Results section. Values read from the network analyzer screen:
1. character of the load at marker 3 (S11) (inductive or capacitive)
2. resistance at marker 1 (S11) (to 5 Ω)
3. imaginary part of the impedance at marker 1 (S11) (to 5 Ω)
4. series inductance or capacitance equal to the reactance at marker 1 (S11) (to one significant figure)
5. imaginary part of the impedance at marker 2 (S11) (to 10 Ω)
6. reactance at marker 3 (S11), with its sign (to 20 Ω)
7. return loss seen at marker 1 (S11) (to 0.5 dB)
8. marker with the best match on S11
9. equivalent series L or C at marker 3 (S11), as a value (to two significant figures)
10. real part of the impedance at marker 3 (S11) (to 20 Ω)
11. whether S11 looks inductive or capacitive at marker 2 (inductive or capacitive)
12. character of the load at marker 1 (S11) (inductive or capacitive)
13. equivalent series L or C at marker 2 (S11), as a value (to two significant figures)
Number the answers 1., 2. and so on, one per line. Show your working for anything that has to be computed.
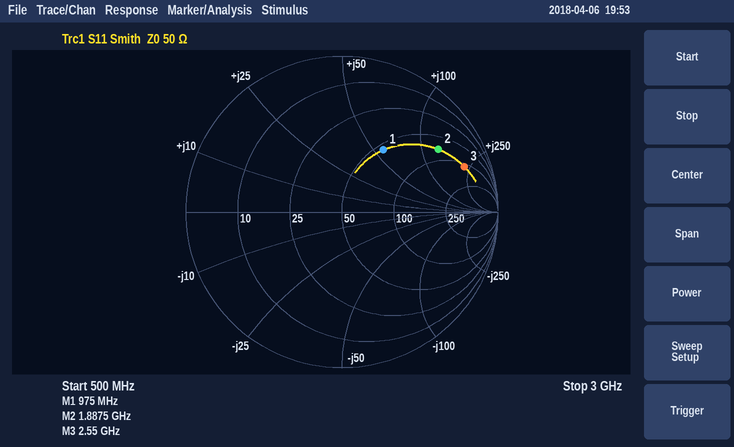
1. inductive
2. 55 Ω
3. +55 Ω
4. L = 55 Ω/(2π × 975 MHz) ≈ 9 nH
5. +130 Ω
6. +220 Ω
7. 6.5 dB
8. marker 1
9. L = 220 Ω/(2π × 2.55 GHz) ≈ 14 nH
10. 120 Ω
11. inductive
12. inductive
13. L = 130 Ω/(2π × 1.8875 GHz) ≈ 11 nH
